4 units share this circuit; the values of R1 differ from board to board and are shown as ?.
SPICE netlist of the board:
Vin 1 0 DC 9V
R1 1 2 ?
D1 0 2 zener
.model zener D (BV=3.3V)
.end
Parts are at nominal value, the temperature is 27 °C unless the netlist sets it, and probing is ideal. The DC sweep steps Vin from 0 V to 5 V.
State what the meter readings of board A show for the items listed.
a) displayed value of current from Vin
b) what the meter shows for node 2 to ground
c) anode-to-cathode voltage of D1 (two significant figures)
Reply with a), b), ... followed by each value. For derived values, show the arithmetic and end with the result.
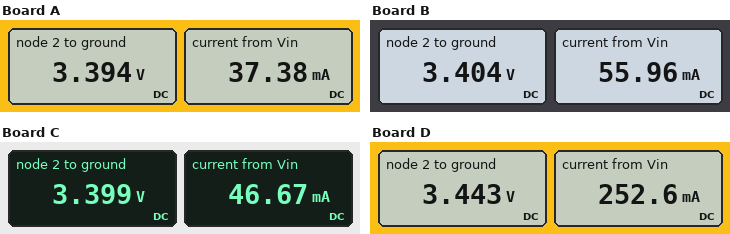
a) 37.38 mA
b) 3.394 V
c) 0 V - 3.394 V = -3.4 V
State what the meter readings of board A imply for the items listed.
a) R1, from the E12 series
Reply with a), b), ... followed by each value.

a) 150 Ω
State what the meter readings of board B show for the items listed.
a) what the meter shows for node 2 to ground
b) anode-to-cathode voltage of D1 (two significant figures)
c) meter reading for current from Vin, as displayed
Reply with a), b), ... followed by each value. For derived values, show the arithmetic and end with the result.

a) 3.404 V
b) 0 V - 3.404 V = -3.4 V
c) 55.96 mA
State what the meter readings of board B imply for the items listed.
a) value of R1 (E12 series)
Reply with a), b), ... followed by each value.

a) 100 Ω
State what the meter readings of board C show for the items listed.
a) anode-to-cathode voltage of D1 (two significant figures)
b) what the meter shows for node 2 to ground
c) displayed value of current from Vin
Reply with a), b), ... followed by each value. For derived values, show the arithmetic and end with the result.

a) 0 V - 3.399 V = -3.4 V
b) 3.399 V
c) 46.67 mA
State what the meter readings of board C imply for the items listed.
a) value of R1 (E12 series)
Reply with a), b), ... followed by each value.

a) 120 Ω
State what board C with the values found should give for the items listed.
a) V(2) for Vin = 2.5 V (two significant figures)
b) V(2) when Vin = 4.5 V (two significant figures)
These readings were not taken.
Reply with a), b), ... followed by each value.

a) 2.5 V
b) 3.4 V
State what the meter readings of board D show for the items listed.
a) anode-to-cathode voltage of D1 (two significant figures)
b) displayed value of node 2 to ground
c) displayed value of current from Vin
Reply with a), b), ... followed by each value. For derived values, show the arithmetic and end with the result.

a) 0 V - 3.443 V = -3.4 V
b) 3.443 V
c) 252.6 mA
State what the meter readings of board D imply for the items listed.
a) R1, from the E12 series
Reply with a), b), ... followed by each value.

a) 22 Ω
